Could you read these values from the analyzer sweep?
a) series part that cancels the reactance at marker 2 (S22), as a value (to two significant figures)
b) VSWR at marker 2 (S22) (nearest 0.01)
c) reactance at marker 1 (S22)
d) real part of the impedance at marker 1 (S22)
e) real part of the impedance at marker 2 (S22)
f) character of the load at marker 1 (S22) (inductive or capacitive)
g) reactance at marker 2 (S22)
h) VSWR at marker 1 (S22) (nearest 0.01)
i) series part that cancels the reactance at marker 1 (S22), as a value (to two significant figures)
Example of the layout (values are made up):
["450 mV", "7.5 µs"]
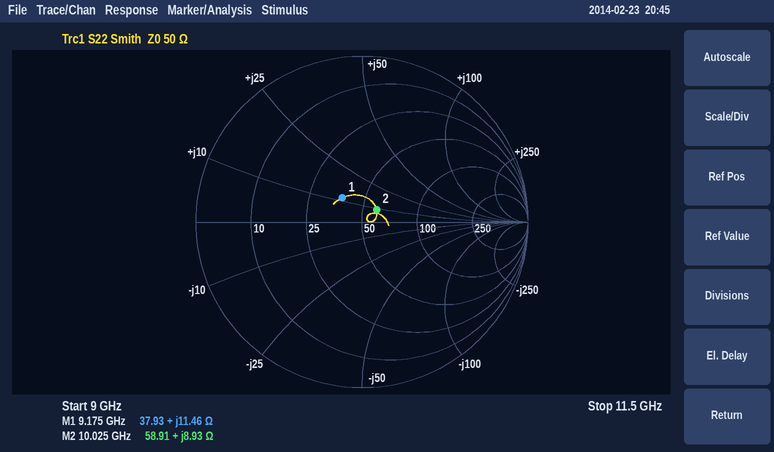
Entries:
["1.8 pF", "1.26", "+11.46 Ω", "37.93 Ω", "58.91 Ω", "inductive", "+8.93 Ω", "1.46", "1.5 pF"]
